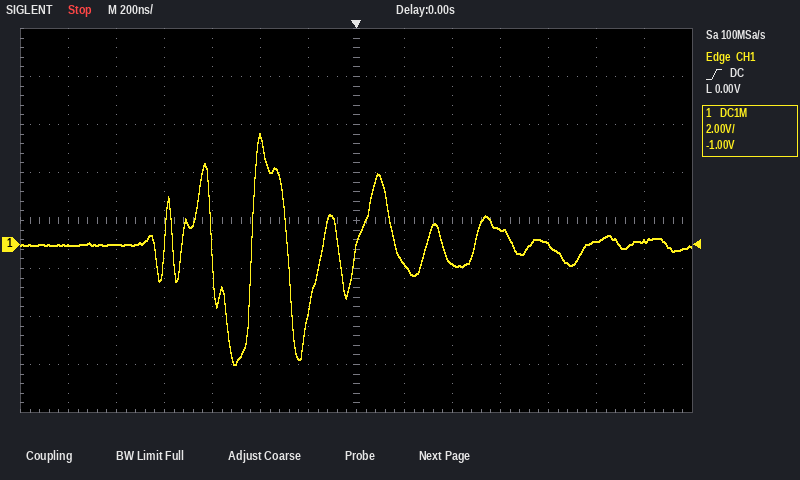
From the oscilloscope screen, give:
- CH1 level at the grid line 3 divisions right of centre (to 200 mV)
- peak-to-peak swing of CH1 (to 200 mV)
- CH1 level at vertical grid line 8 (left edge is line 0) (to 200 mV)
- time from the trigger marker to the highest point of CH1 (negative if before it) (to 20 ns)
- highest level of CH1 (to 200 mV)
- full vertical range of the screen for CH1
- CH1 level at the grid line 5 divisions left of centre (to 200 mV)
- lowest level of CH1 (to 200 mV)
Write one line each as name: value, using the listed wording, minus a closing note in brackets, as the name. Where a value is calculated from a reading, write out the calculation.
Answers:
CH1 level at the grid line 3 divisions right of centre: 600 mV
peak-to-peak swing of CH1: 4.6 V − (-5.0 V) = 9.6 V
CH1 level at vertical grid line 8 (left edge is line 0): -800 mV
time from the trigger marker to the highest point of CH1 (negative if before it): -400 ns
highest level of CH1: 4.6 V
full vertical range of the screen for CH1: 16 V
CH1 level at the grid line 5 divisions left of centre: 0.0 V
lowest level of CH1: -5.0 V
